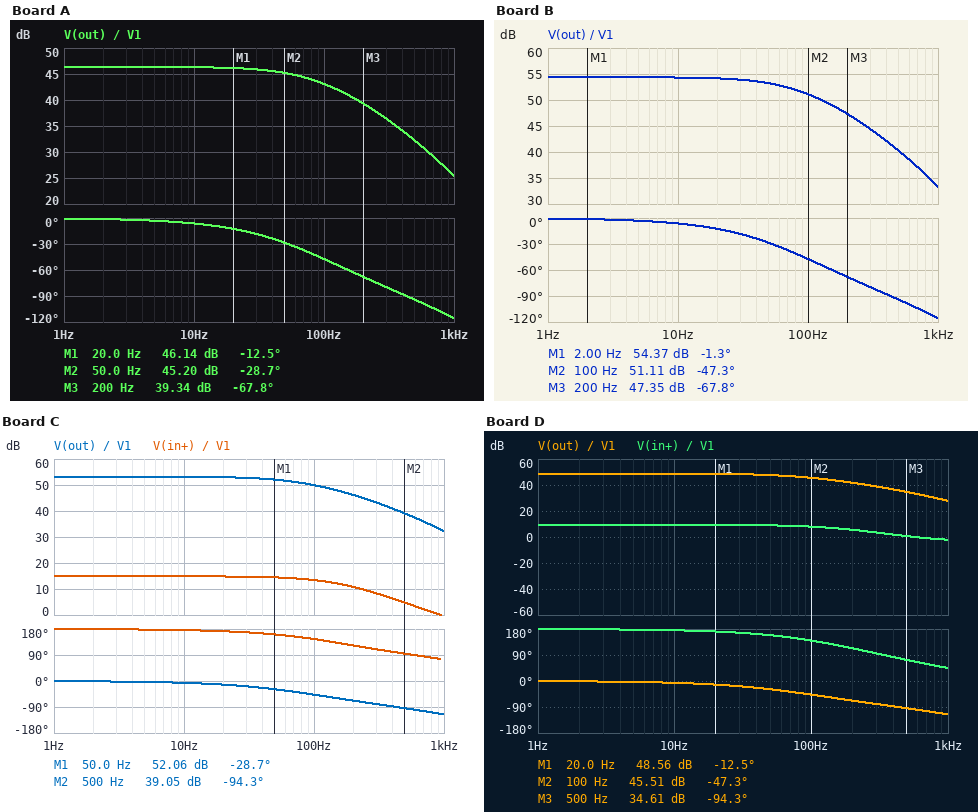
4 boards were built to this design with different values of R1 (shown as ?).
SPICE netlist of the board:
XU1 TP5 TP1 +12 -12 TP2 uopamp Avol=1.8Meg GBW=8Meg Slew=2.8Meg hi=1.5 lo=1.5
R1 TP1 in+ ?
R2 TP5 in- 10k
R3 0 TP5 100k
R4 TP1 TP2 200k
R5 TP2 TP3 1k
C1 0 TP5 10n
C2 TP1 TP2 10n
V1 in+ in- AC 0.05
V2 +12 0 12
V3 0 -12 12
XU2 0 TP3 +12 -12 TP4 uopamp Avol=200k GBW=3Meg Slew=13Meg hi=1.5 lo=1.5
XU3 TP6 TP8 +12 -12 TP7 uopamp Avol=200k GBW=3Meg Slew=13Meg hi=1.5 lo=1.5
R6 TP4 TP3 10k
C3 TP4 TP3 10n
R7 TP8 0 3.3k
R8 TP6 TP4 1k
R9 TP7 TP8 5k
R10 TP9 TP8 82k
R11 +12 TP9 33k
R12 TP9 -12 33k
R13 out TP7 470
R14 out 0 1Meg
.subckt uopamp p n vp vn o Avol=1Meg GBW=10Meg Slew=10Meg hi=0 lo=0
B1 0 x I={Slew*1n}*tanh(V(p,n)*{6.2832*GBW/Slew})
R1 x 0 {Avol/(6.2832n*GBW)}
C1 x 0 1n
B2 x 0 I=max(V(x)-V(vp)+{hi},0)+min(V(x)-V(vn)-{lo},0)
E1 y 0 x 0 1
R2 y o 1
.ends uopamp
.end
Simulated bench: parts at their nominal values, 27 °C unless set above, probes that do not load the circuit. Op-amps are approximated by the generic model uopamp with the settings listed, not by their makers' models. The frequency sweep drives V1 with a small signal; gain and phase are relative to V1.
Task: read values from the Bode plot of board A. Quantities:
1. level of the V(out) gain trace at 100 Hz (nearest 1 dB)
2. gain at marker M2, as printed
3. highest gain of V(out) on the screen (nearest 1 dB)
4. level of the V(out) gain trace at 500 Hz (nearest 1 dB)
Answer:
43 dB
45.20 dB
46 dB
32 dB
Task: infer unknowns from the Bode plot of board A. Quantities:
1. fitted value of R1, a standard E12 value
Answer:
27 kΩ
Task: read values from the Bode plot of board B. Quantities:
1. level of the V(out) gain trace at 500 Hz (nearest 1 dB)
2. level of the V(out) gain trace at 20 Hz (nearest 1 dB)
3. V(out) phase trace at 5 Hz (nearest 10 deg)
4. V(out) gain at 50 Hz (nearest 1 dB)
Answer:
40 dB
54 dB
0 deg
53 dB
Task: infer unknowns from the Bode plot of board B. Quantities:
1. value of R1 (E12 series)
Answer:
4.7 kΩ
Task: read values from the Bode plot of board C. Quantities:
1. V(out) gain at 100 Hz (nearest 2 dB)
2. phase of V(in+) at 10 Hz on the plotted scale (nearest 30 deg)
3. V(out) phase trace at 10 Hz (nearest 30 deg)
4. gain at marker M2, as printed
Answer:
50 dB
180 deg
0 deg
39.05 dB
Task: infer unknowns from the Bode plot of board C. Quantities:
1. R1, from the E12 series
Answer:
6.8 kΩ
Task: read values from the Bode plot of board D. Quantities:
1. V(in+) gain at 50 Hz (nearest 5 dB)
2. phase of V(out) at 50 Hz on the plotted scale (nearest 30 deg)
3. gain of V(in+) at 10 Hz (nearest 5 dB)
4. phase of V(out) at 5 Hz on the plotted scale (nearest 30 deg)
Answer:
10 dB
-30 deg
10 dB
0 deg
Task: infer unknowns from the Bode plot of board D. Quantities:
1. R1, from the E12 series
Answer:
18 kΩ
